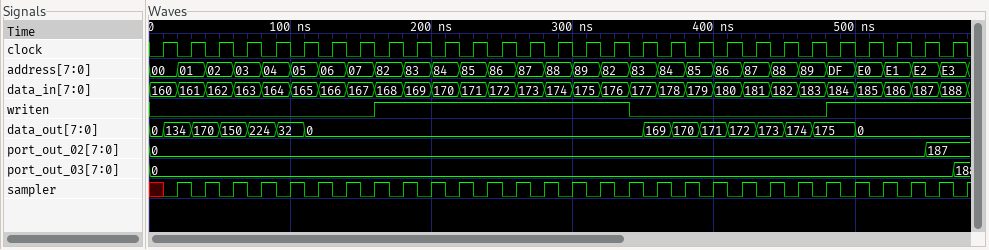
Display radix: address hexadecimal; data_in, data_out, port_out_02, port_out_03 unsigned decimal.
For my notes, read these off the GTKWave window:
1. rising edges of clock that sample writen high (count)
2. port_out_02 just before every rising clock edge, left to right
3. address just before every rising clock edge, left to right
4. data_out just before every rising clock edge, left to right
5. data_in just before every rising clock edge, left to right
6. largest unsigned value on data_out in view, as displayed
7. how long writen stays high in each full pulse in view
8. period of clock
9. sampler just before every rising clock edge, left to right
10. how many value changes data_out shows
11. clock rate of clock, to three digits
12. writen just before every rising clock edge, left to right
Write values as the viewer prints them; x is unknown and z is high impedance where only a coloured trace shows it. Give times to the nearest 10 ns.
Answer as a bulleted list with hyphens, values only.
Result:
- 14
- 0, 0, 0, 0, 0, 0, 0, 0, 0, 0, 0, 0, 0, 0, 0, 0, 0, 0, 0, 0, 0, 0, 0, 0, 0, 0, 0, 0, 187
- 00, 01, 02, 03, 04, 05, 06, 07, 82, 83, 84, 85, 86, 87, 88, 89, 82, 83, 84, 85, 86, 87, 88, 89, DF, E0, E1, E2, E3
- 0, 134, 170, 150, 224, 32, 0, 0, 0, 0, 0, 0, 0, 0, 0, 0, 0, 0, 169, 170, 171, 172, 173, 174, 175, 0, 0, 0, 0
- 160, 161, 162, 163, 164, 165, 166, 167, 168, 169, 170, 171, 172, 173, 174, 175, 176, 177, 178, 179, 180, 181, 182, 183, 184, 185, 186, 187, 188
- 224
- 180 ns
- 20 ns
- x 1 1 1 1 1 1 1 1 1 1 1 1 1 1 1 1 1 1 1 1 1 1 1 1 1 1 1 1
- 14
- 50.0 MHz
- 0 0 0 0 0 0 0 0 1 1 1 1 1 1 1 1 1 0 0 0 0 0 0 0 1 1 1 1 1
